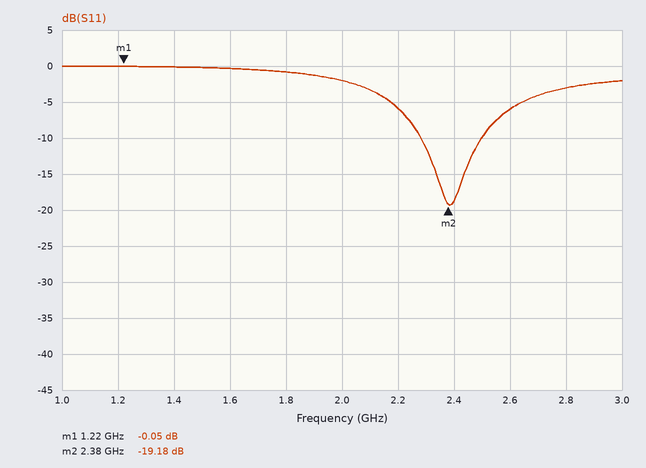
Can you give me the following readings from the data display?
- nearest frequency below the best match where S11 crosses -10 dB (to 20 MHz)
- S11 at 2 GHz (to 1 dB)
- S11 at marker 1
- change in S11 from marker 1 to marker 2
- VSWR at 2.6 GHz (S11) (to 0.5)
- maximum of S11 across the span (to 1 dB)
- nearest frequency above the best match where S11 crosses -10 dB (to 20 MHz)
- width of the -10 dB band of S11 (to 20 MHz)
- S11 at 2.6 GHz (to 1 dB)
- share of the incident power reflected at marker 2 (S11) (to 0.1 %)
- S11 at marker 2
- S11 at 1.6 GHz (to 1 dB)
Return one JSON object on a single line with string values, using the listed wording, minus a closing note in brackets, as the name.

{"nearest frequency below the best match where S11 crosses -10 dB": "2.28 GHz", "S11 at 2 GHz": "-2 dB", "S11 at marker 1": "-0.05 dB", "change in S11 from marker 1 to marker 2": "-19.13 dB", "VSWR at 2.6 GHz (S11)": "3.0", "maximum of S11 across the span": "0 dB", "nearest frequency above the best match where S11 crosses -10 dB": "2.50 GHz", "width of the -10 dB band of S11": "220 MHz", "S11 at 2.6 GHz": "-6 dB", "share of the incident power reflected at marker 2 (S11)": "1.2 %", "S11 at marker 2": "-19.18 dB", "S11 at 1.6 GHz": "0 dB"}
